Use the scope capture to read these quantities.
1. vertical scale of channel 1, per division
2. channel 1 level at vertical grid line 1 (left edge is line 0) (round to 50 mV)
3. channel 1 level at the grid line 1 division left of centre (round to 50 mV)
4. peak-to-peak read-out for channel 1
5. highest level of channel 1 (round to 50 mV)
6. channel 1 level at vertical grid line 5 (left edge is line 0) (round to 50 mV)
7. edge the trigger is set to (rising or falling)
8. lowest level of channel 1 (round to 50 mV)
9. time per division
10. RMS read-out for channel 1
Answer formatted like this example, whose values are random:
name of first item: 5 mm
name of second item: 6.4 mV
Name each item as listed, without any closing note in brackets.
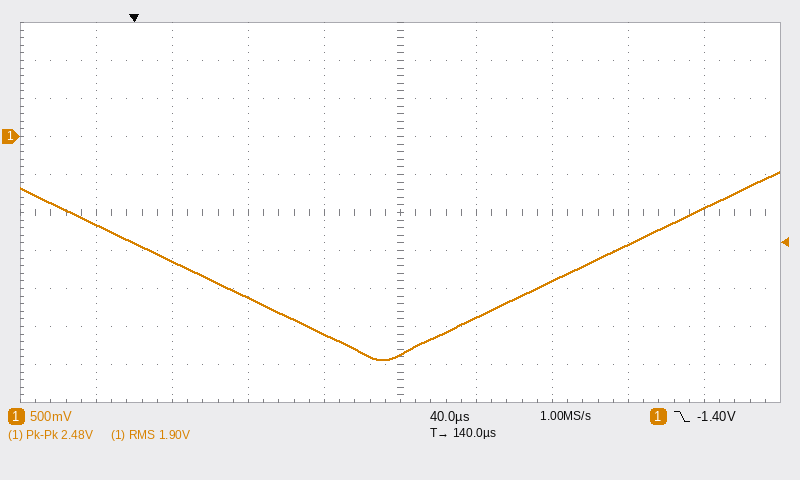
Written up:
vertical scale of channel 1, per division: 500 mV
channel 1 level at vertical grid line 1 (left edge is line 0): -1.15 V
channel 1 level at the grid line 1 division left of centre: -2.60 V
peak-to-peak read-out for channel 1: 2.48 V
highest level of channel 1: -450 mV
channel 1 level at vertical grid line 5 (left edge is line 0): -2.85 V
edge the trigger is set to: falling
lowest level of channel 1: -2.95 V
time per division: 40 µs
RMS read-out for channel 1: 1.90 V
